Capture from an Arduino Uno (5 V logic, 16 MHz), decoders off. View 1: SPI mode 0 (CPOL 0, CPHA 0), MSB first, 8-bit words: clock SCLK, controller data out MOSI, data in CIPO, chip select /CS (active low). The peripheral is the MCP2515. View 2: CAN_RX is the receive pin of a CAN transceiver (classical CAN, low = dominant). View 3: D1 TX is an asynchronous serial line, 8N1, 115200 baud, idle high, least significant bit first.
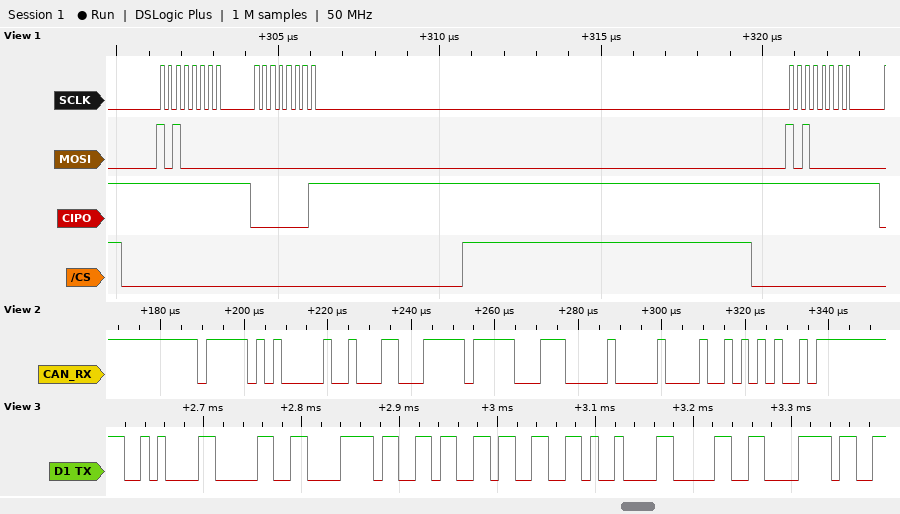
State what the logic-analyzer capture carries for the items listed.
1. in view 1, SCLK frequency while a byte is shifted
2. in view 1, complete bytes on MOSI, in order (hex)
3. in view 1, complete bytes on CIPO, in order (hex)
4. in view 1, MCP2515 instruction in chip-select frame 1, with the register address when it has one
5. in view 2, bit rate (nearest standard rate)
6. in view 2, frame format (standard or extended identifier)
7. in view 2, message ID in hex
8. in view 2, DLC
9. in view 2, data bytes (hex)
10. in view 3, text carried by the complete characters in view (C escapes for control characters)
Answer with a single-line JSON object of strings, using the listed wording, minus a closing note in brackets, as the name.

{"in view 1, SCLK frequency while a byte is shifted": "4 MHz", "in view 1, complete bytes on MOSI, in order": "0xA0 0x00 0xA0", "in view 1, complete bytes on CIPO, in order": "0xFF 0x01 0xFF", "in view 1, MCP2515 instruction in chip-select frame 1, with the register address when it has one": "READ STATUS", "in view 2, bit rate": "500 kbit/s", "in view 2, frame format": "standard", "in view 2, message ID in hex": "0x7E8", "in view 2, DLC": "4", "in view 2, data bytes": "63 FF 38 00", "in view 3, text carried by the complete characters in view": "\"\\n0x63\\t0x\""}
